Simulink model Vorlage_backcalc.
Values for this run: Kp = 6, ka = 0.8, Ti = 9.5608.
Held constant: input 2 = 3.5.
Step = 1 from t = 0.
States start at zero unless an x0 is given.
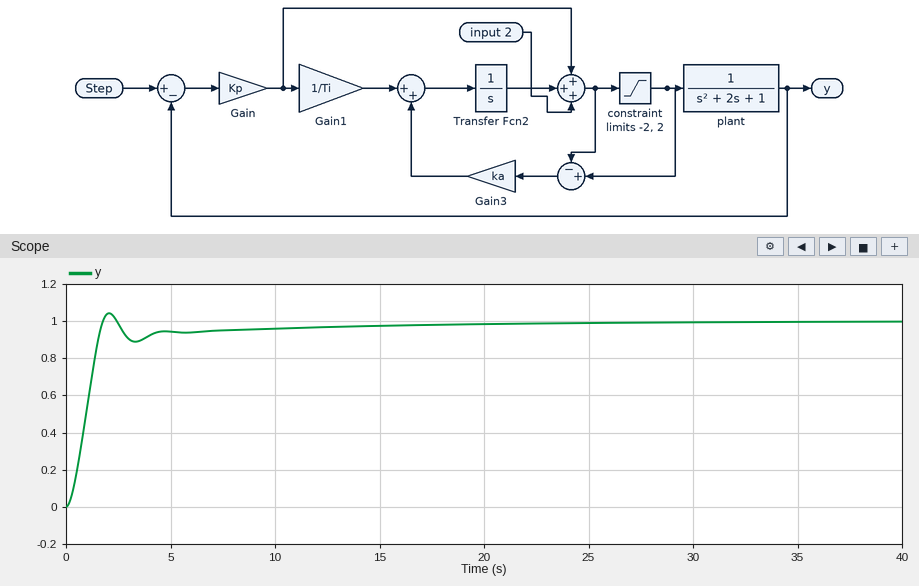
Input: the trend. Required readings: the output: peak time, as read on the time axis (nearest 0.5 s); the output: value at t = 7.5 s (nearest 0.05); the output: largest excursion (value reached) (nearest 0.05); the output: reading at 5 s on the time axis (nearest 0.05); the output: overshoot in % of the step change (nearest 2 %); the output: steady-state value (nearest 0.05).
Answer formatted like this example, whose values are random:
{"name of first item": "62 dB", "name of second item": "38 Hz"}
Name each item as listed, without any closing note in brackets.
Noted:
{"the output: peak time, as read on the time axis": "2.0 s", "the output: value at t = 7.5 s": "0.95", "the output: largest excursion (value reached)": "1.05", "the output: reading at 5 s on the time axis": "0.95", "the output: overshoot in % of the step change": "4 %", "the output: steady-state value": "1.00"}
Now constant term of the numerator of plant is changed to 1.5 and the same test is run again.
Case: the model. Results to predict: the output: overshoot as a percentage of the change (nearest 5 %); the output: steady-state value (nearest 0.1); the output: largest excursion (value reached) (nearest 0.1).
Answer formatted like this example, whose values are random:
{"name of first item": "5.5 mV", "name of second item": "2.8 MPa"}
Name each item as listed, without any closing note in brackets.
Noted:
{"the output: overshoot as a percentage of the change": "20 %", "the output: steady-state value": "1.0", "the output: largest excursion (value reached)": "1.2"}
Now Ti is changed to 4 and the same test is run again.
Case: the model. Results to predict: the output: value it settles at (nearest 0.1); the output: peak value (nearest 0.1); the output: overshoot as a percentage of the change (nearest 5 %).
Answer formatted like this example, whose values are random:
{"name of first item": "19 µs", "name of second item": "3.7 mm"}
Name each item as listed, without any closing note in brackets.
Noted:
{"the output: value it settles at": "1.0", "the output: peak value": "1.1", "the output: overshoot as a percentage of the change": "10 %"}
